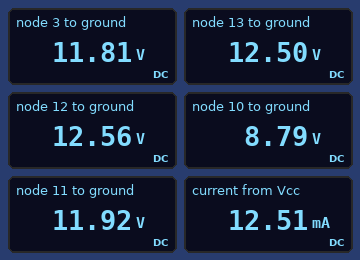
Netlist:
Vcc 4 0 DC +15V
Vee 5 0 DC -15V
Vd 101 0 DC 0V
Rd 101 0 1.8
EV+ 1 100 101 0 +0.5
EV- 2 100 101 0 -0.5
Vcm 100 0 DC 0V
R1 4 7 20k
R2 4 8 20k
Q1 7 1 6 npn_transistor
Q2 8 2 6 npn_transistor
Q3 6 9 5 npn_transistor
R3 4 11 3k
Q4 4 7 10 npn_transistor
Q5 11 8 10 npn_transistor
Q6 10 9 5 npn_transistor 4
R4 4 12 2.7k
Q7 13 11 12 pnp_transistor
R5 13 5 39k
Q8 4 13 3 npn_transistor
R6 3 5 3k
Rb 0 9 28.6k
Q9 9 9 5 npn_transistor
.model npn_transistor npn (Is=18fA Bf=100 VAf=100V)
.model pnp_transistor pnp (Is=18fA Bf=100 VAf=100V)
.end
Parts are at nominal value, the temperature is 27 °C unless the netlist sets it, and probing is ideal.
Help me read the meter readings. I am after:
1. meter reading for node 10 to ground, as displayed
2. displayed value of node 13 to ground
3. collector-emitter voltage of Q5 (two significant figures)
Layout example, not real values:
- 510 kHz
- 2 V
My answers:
- 8.79 V
- 12.50 V
- 3.1 V
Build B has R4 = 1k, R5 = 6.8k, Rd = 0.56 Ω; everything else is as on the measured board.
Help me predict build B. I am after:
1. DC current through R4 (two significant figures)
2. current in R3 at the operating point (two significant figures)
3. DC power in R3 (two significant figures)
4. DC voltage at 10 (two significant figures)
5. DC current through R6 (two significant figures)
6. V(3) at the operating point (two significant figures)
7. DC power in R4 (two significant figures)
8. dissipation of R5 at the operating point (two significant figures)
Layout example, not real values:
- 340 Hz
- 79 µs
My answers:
- 2.7 mA
- 1.1 mA
- 3.7 mW
- 8.8 V
- 5.7 mA
- 2.0 V
- 7.2 mW
- 46 mW
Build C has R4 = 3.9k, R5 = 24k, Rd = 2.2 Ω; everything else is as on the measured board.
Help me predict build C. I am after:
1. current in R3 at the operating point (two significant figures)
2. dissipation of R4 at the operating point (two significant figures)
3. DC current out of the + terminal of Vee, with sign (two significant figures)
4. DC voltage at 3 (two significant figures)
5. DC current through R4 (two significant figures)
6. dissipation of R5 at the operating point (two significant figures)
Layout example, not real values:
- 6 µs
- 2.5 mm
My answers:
- 1.1 mA
- 2.0 mW
- -9.1 mA
- 150 mV
- 710 µA
- 10 mW
